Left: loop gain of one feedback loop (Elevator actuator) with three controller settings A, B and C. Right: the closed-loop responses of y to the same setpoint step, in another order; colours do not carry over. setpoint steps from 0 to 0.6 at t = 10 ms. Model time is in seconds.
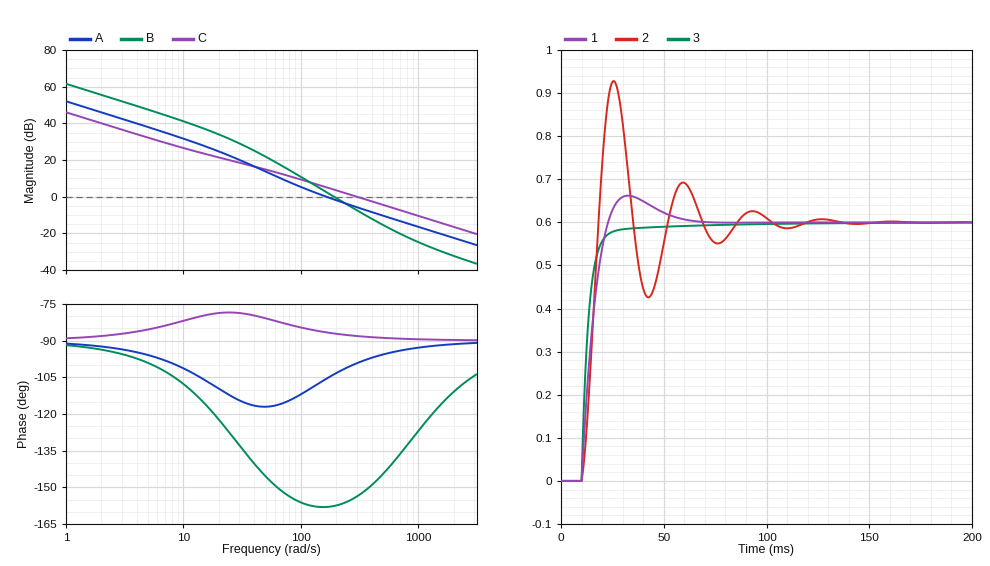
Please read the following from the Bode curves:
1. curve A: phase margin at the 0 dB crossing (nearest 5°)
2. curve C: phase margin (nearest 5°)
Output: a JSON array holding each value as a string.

["75°", "90°"]
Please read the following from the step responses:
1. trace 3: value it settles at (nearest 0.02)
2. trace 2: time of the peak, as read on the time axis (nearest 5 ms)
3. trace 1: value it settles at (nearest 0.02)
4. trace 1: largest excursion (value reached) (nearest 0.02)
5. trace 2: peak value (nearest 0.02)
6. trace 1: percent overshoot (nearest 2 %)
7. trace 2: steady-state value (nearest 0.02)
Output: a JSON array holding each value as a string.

["0.60", "25 ms", "0.60", "0.66", "0.92", "10 %", "0.60"]
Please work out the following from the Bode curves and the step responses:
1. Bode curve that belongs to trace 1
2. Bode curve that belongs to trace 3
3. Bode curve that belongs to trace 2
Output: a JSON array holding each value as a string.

["A", "C", "B"]
